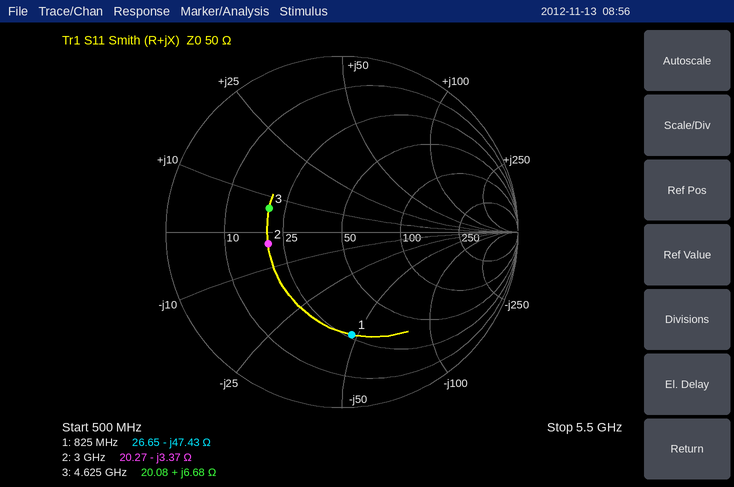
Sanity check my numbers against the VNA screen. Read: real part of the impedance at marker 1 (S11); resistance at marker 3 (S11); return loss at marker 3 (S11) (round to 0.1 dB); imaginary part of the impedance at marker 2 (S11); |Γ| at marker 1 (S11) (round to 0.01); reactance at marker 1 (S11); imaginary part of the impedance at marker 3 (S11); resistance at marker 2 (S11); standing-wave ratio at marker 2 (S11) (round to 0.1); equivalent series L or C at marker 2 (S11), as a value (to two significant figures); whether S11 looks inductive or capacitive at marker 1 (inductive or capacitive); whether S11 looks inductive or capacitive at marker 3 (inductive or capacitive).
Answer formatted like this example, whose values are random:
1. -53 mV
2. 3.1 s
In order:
1. 26.65 Ω
2. 20.08 Ω
3. 7.2 dB
4. -3.37 Ω
5. 0.59
6. -47.43 Ω
7. +6.68 Ω
8. 20.27 Ω
9. 2.5
10. 16 pF
11. capacitive
12. inductive
